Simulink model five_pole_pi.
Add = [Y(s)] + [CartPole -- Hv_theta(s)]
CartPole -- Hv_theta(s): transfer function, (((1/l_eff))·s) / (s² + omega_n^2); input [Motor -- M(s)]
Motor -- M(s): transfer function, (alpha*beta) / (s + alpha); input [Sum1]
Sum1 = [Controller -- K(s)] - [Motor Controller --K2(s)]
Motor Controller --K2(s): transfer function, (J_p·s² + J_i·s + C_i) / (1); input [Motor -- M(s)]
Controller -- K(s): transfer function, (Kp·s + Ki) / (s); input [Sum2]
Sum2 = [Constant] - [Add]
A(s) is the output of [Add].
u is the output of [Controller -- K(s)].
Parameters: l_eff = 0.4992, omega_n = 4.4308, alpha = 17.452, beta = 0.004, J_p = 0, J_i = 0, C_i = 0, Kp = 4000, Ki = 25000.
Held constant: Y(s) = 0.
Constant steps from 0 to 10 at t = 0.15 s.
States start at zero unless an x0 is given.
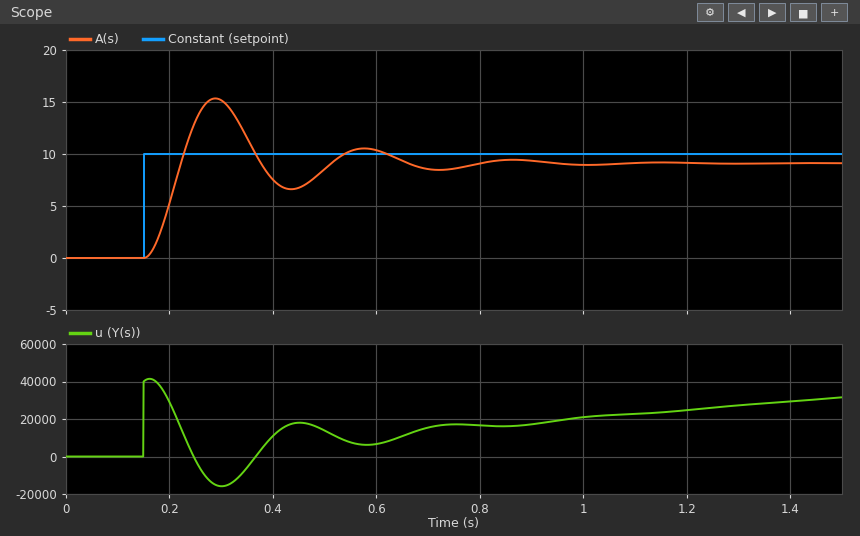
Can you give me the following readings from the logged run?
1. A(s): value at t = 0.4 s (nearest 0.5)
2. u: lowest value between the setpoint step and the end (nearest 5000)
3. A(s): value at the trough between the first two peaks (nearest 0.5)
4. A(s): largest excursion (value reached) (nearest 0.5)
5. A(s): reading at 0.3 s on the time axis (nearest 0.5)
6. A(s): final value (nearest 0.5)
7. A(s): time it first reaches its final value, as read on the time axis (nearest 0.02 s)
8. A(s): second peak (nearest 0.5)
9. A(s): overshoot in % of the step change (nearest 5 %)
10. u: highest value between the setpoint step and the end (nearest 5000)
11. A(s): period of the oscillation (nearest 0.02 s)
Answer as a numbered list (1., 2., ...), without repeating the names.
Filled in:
1. 7.5
2. -15000
3. 6.5
4. 15.5
5. 15.0
6. 9.0
7. 0.22 s
8. 10.5
9. 70 %
10. 40000
11. 0.28 s
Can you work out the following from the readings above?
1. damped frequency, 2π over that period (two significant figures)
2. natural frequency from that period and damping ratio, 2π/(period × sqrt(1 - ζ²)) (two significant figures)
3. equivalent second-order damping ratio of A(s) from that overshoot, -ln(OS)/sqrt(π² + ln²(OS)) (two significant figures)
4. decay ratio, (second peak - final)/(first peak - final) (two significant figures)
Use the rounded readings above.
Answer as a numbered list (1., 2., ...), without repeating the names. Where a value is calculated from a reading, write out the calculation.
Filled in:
1. 2π / 0.28 = 22 rad/s
2. 2π / (0.28 × sqrt(1 - 0.11²)) = 23 rad/s
3. ln(0.7) = -0.357; 0.357 / sqrt(9.870 + 0.127) = 0.11
4. (10.5 - 9) / (15.5 - 9) = 0.23
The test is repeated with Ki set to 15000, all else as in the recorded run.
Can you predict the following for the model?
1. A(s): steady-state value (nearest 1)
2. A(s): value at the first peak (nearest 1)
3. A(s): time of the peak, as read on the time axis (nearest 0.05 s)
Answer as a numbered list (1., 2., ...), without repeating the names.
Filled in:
1. 9
2. 14
3. 0.30 s
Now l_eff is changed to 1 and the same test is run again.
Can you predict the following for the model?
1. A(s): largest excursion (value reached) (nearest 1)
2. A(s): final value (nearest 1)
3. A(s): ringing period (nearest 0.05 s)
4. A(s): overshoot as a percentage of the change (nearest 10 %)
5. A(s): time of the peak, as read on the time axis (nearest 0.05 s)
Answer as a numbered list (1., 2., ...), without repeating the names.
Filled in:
1. 14
2. 8
3. 0.45 s
4. 70 %
5. 0.35 s
